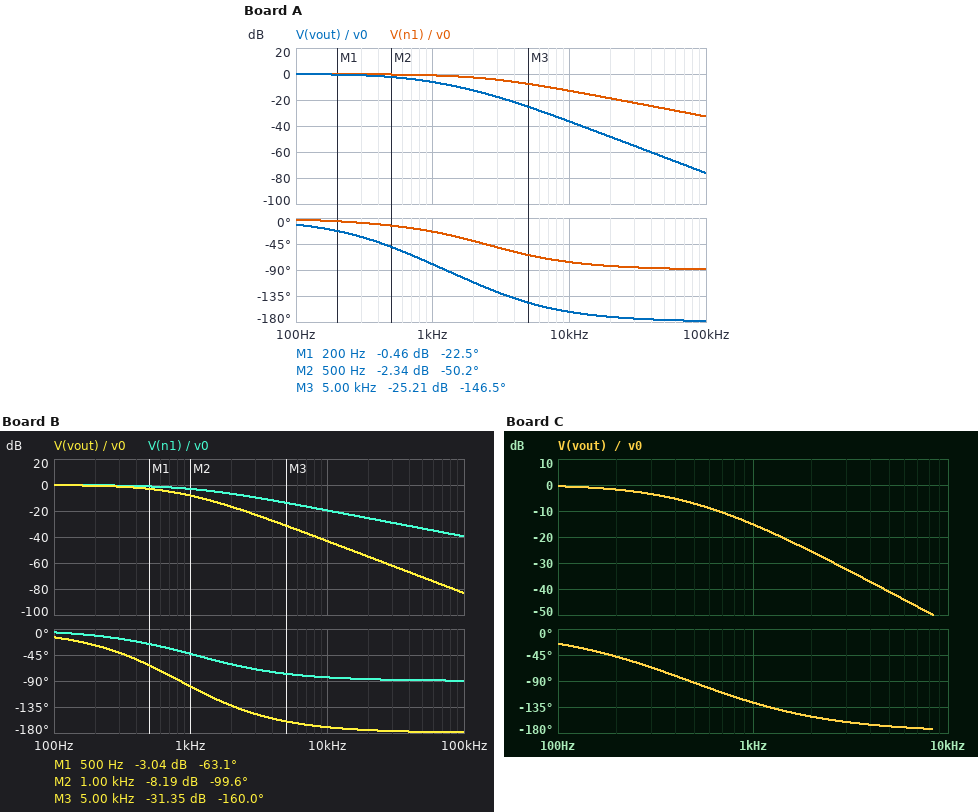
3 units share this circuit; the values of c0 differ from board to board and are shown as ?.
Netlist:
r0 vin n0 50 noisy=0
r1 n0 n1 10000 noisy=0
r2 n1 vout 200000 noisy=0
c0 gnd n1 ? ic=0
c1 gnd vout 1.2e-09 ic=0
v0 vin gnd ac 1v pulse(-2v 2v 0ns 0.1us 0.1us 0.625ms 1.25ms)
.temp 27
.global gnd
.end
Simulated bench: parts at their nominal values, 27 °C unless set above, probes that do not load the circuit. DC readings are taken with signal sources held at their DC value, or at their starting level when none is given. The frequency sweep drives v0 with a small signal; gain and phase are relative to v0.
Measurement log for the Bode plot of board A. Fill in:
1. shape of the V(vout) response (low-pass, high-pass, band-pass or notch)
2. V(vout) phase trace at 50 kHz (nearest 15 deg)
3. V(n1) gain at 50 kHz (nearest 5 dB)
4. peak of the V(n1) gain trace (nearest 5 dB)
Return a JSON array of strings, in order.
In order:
["low-pass", "-180 deg", "-25 dB", "0 dB"]
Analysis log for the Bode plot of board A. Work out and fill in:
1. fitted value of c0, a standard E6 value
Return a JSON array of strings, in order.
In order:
["6.8 nF"]
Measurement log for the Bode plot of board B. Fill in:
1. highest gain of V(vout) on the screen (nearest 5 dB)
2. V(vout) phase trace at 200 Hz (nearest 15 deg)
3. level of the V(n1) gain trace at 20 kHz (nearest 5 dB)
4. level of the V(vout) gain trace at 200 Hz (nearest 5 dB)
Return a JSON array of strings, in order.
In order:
["0 dB", "-30 deg", "-25 dB", "0 dB"]
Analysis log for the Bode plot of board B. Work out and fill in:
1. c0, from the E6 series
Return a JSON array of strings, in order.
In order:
["15 nF"]
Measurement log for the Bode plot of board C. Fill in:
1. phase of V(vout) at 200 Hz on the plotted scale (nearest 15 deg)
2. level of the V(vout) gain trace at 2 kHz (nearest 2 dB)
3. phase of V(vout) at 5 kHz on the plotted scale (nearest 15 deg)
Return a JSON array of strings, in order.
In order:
["-45 deg", "-26 dB", "-165 deg"]
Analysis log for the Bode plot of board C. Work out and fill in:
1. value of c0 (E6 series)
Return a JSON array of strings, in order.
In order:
["47 nF"]
